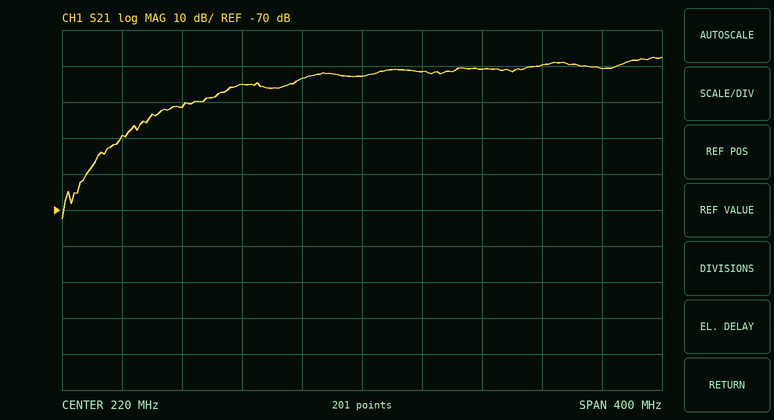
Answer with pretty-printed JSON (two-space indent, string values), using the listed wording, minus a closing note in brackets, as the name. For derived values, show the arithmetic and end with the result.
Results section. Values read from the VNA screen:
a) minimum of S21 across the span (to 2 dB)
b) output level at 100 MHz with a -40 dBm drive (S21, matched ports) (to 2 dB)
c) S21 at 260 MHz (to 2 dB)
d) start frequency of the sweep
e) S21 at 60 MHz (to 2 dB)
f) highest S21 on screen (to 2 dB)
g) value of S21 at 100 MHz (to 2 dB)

{
  "minimum of S21 across the span": "-72 dB",
  "output level at 100 MHz with a -40 dBm drive (S21, matched ports)": "-40 dBm + (-42 dB) = -82 dBm",
  "S21 at 260 MHz": "-32 dB",
  "start frequency of the sweep": "20 MHz",
  "S21 at 60 MHz": "-50 dB",
  "highest S21 on screen": "-28 dB",
  "value of S21 at 100 MHz": "-42 dB"
}
